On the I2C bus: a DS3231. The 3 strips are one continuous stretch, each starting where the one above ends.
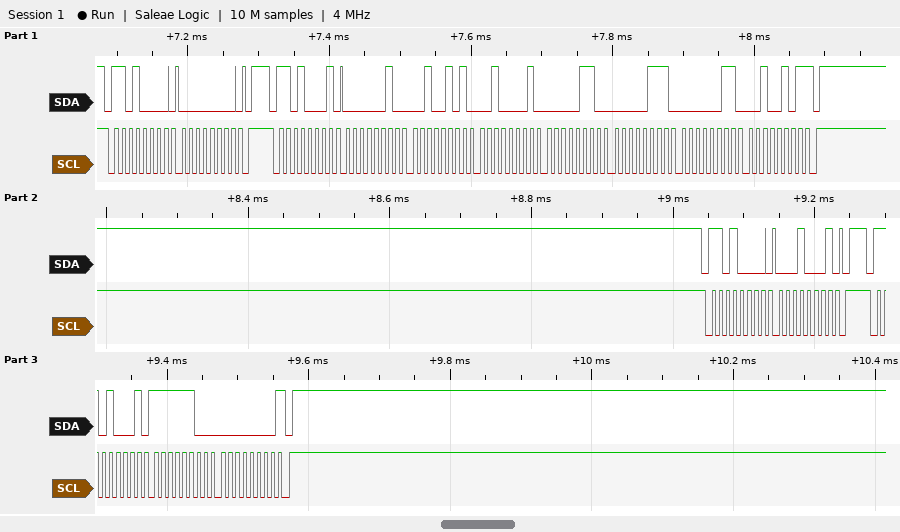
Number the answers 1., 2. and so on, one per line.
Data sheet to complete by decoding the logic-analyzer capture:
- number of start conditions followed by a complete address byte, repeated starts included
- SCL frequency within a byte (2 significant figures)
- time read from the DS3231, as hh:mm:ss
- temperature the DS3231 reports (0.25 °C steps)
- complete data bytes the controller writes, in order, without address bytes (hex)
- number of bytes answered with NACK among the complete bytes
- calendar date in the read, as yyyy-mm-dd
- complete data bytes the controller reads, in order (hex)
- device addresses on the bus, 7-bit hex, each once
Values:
1. 4
2. 100 kHz
3. 21:25:02
4. -4.00 °C
5. 00 11
6. 2
7. 2025-03-07
8. 02 25 21 06 07 03 25 FC 00
9. 0x68
